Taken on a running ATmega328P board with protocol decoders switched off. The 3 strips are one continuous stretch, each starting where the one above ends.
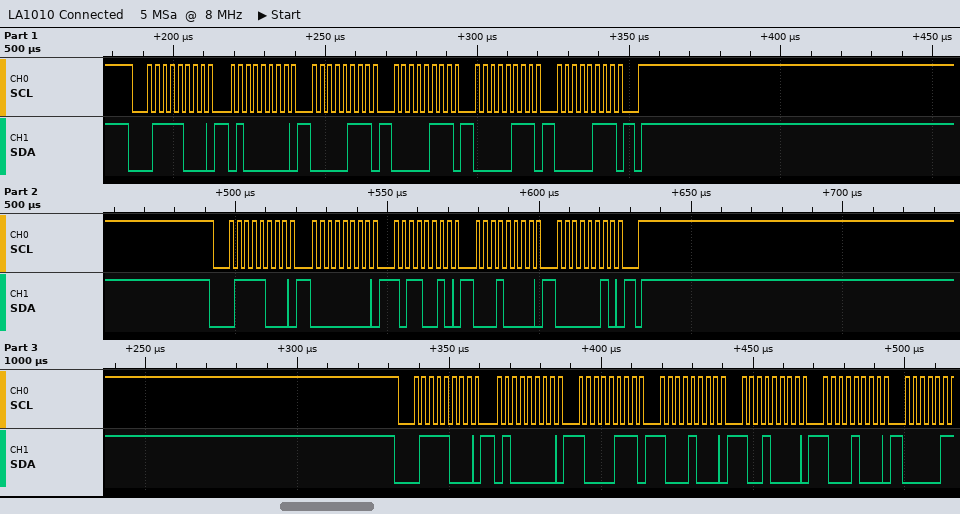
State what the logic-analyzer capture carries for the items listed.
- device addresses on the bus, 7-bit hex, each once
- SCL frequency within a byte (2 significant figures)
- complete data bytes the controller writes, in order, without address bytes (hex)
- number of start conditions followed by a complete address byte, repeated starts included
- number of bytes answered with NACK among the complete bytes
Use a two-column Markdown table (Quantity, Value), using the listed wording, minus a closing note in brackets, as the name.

| Quantity | Value |
|---|---|
| device addresses on the bus, 7-bit hex, each once | 0x3C |
| SCL frequency within a byte | 400 kHz |
| complete data bytes the controller writes, in order, without address bytes | 40 07 07 07 07 00 B2 10 02 40 87 88 90 88 |
| number of start conditions followed by a complete address byte, repeated starts included | 3 |
| number of bytes answered with NACK among the complete bytes | 0 |
